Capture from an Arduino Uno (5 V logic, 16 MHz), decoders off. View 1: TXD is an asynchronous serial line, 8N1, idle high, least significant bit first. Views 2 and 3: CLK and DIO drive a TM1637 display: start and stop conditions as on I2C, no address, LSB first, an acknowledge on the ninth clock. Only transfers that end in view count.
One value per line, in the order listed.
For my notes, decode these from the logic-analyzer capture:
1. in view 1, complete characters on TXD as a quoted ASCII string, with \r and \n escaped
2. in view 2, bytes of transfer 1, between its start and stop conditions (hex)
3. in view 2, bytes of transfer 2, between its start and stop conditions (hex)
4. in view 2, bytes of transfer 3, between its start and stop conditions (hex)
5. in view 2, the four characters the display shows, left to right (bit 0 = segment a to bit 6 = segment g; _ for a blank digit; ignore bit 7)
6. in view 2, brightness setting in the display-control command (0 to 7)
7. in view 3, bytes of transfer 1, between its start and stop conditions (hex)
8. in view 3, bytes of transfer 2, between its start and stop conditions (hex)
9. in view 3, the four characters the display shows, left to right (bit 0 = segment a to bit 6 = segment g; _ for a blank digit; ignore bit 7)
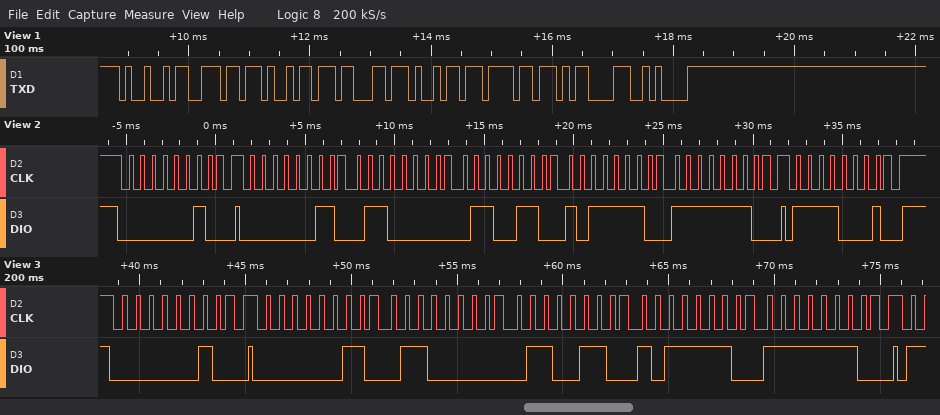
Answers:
"Inicio\r\n"
40
C0 06 66 7D 7F
8F
1468
7
40
C0 06 66 7D 7F
1468
